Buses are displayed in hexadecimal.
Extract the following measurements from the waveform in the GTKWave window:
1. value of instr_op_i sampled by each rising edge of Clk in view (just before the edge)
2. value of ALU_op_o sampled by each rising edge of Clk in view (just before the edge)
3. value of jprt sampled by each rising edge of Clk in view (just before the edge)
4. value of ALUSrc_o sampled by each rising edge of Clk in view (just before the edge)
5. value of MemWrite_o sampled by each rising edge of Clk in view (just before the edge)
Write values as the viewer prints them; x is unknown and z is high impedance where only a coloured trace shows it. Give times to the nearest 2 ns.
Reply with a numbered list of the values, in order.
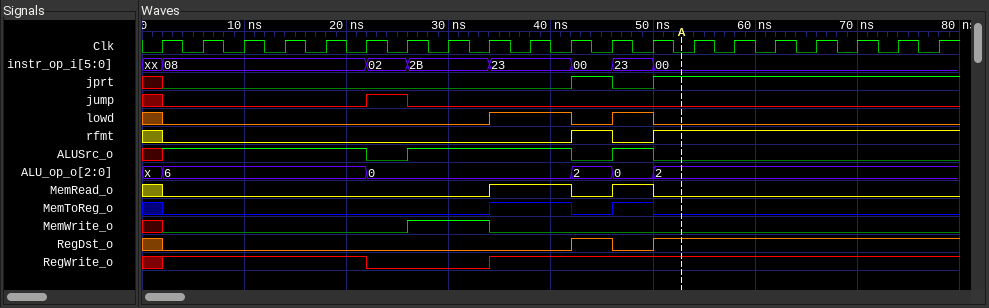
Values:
1. xx, 08, 08, 08, 08, 08, 02, 2B, 2B, 23, 23, 00, 23, 00, 00, 00, 00, 00, 00, 00
2. x, 6, 6, 6, 6, 6, 0, 0, 0, 0, 0, 2, 0, 2, 2, 2, 2, 2, 2, 2
3. x 0 0 0 0 0 0 0 0 0 0 1 0 1 1 1 1 1 1 1
4. x 1 1 1 1 1 0 1 1 1 1 0 1 0 0 0 0 0 0 0
5. x 0 0 0 0 0 0 1 1 0 0 0 0 0 0 0 0 0 0 0
